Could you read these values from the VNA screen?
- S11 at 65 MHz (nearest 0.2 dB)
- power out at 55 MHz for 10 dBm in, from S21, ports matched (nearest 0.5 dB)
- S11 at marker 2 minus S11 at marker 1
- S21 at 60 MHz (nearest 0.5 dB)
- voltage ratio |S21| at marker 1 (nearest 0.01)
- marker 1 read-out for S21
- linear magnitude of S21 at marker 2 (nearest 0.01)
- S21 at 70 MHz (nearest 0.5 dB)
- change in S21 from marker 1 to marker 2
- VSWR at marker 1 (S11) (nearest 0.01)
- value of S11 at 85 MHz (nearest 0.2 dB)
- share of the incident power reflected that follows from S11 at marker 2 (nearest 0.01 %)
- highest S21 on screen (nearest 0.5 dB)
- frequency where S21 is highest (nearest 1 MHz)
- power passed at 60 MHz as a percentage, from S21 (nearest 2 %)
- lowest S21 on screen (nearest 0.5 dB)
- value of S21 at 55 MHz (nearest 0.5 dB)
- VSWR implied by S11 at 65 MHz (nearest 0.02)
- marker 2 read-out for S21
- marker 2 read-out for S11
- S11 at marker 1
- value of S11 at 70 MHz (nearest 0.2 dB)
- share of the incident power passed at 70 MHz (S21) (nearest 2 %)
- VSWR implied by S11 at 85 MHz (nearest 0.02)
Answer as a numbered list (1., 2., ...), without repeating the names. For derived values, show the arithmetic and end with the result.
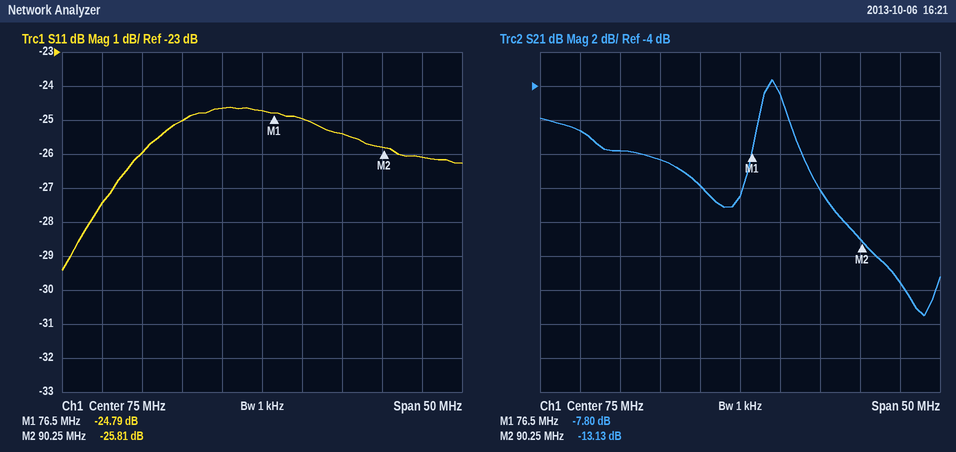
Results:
1. -25.0 dB
2. 10 dBm + (-6.5 dB) = 3.5 dBm
3. -25.81 − (-24.79) = -1.02 dB
4. -8.0 dB
5. 10^(-7.8/20) ≈ 0.41
6. -7.80 dB
7. 10^(-13.13/20) ≈ 0.22
8. -10.0 dB
9. -13.13 − (-7.8) = -5.33 dB
10. (1 + 0.0576)/(1 − 0.0576) ≈ 1.12
11. -25.4 dB
12. 10^(-25.81/10) ≈ 0.26 %
13. -3.5 dB
14. 79 MHz
15. 10^(-8/10) ≈ 16 %
16. -17.5 dB
17. -6.5 dB
18. |Γ| = 10^(-25/20) = 0.0562; VSWR = (1 + 0.0562)/(1 − 0.0562) ≈ 1.12
19. -13.13 dB
20. -25.81 dB
21. -24.79 dB
22. -24.6 dB
23. 10^(-10/10) ≈ 10 %
24. |Γ| = 10^(-25.4/20) = 0.0537; VSWR = (1 + 0.0537)/(1 − 0.0537) ≈ 1.11, so 1.12 to the nearest 0.02
